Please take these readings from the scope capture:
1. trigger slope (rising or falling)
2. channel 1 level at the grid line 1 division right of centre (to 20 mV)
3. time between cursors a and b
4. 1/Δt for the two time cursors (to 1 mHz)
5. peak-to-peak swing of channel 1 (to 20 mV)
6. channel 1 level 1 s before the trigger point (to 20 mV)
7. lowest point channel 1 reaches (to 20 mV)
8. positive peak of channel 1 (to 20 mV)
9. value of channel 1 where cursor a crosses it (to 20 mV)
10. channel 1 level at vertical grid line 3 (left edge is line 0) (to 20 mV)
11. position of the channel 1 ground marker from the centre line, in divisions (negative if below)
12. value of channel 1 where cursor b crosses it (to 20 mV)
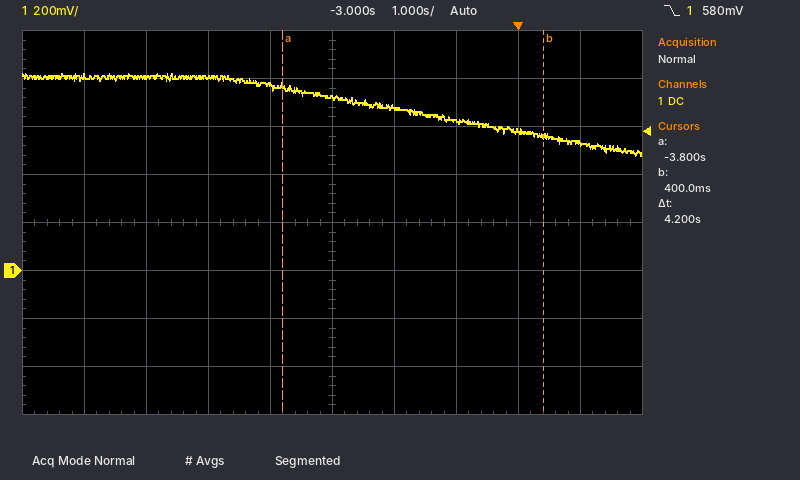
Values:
falling
680 mV
4.2 s
238 mHz
340 mV
620 mV
480 mV
820 mV
760 mV
800 mV
-1.0 div
560 mV
